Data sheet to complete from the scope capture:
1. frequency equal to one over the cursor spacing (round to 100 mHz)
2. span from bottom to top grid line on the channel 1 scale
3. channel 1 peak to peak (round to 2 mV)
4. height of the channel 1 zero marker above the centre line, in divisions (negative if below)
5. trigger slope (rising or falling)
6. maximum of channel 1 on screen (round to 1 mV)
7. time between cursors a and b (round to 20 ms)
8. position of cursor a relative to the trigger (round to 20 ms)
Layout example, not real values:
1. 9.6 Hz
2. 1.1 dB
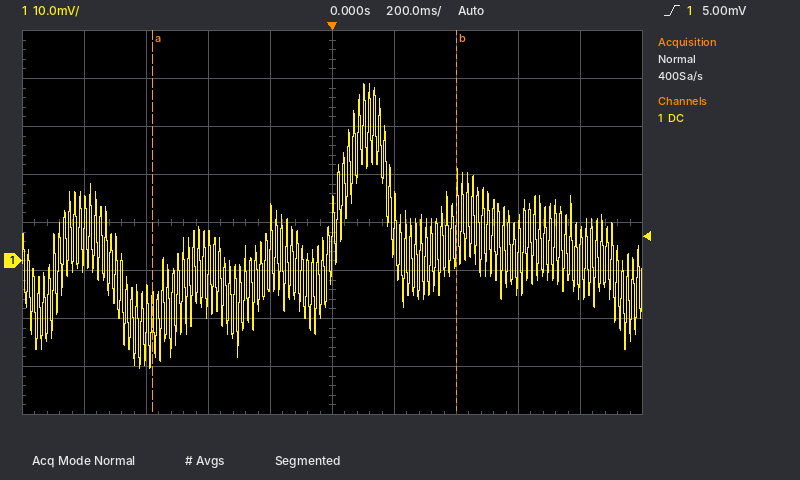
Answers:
1. 1.0 Hz
2. 80 mV
3. 60 mV
4. -0.8 div
5. rising
6. 37 mV
7. 980 ms
8. -580 ms
